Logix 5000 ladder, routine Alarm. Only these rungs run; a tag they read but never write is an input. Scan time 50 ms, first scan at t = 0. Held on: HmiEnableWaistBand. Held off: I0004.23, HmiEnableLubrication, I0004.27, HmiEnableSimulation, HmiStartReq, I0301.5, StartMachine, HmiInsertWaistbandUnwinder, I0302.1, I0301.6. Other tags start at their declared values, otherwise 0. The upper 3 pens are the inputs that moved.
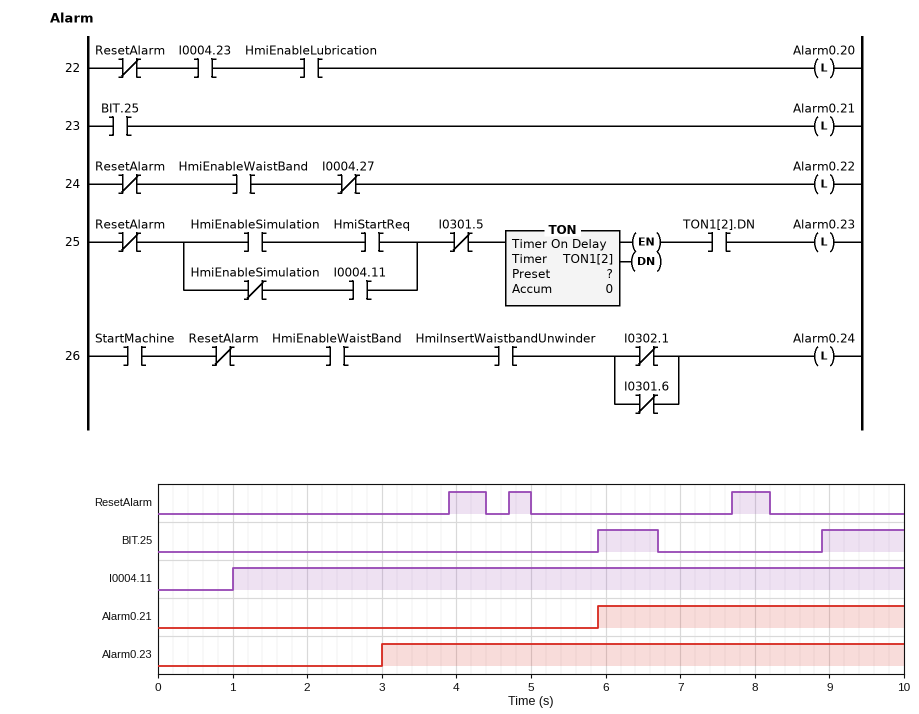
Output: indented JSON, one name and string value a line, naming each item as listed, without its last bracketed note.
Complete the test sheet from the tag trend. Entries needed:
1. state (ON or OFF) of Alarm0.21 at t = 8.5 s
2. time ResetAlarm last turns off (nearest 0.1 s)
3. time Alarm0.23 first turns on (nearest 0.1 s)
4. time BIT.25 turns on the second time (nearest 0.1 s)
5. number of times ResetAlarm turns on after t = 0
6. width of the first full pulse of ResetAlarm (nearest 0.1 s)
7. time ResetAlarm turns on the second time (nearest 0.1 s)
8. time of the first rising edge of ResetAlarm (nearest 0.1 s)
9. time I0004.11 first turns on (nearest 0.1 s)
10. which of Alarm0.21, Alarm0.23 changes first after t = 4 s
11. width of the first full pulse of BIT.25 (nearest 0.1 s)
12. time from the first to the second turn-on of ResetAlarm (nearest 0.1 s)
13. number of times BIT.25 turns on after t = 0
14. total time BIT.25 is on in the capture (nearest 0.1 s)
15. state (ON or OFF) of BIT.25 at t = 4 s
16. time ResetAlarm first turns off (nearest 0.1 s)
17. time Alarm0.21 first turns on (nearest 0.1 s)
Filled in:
{
  "state (ON or OFF) of Alarm0.21 at t = 8.5 s": "ON",
  "time ResetAlarm last turns off": "8.2 s",
  "time Alarm0.23 first turns on": "3.0 s",
  "time BIT.25 turns on the second time": "8.9 s",
  "number of times ResetAlarm turns on after t = 0": "3",
  "width of the first full pulse of ResetAlarm": "0.5 s",
  "time ResetAlarm turns on the second time": "4.7 s",
  "time of the first rising edge of ResetAlarm": "3.9 s",
  "time I0004.11 first turns on": "1.0 s",
  "which of Alarm0.21, Alarm0.23 changes first after t = 4 s": "Alarm0.21",
  "width of the first full pulse of BIT.25": "0.8 s",
  "time from the first to the second turn-on of ResetAlarm": "0.8 s",
  "number of times BIT.25 turns on after t = 0": "2",
  "total time BIT.25 is on in the capture": "1.9 s",
  "state (ON or OFF) of BIT.25 at t = 4 s": "OFF",
  "time ResetAlarm first turns off": "4.4 s",
  "time Alarm0.21 first turns on": "5.9 s"
}
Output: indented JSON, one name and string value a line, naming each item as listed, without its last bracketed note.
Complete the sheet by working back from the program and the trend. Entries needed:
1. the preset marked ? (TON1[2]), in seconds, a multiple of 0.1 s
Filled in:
{
  "the preset marked ? (TON1[2]), in seconds, a multiple of 0.1 s": "2.0 s"
}
